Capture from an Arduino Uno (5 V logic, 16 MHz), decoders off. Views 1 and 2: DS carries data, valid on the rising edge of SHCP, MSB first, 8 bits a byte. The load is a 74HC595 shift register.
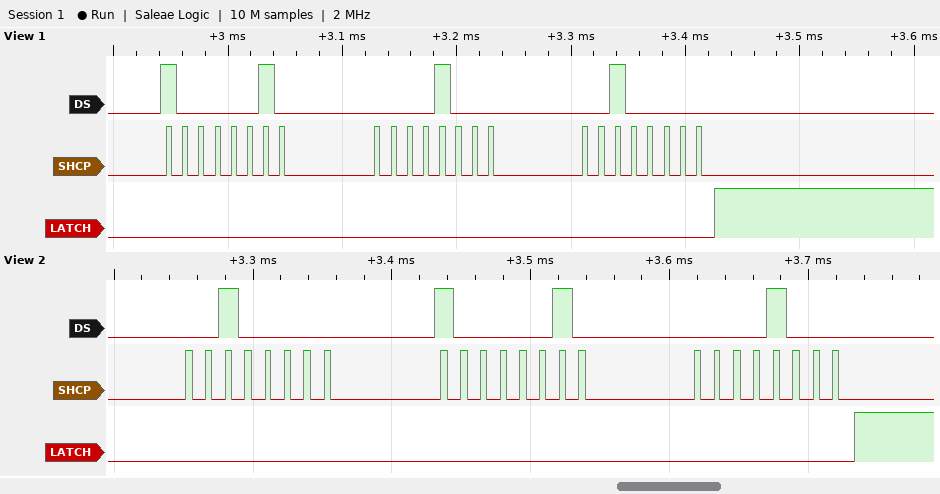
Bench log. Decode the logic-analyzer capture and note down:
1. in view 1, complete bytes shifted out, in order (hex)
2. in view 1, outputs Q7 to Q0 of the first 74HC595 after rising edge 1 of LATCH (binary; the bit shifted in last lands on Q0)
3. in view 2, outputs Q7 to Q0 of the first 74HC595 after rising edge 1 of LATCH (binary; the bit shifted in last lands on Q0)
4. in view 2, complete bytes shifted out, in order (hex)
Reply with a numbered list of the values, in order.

1. 82 08 20
2. 00100000
3. 00001000
4. 20 82 08
